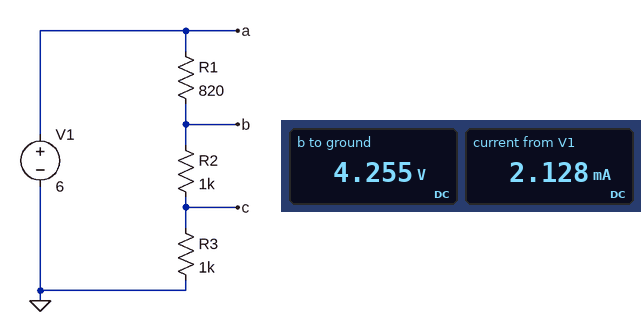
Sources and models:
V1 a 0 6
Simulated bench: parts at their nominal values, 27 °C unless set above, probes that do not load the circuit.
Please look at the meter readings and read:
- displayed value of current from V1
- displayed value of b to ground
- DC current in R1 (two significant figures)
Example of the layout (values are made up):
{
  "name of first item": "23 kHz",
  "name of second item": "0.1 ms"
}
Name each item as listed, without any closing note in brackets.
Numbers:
{
  "displayed value of current from V1": "2.128 mA",
  "displayed value of b to ground": "4.255 V",
  "DC current in R1": "2.1 mA"
}
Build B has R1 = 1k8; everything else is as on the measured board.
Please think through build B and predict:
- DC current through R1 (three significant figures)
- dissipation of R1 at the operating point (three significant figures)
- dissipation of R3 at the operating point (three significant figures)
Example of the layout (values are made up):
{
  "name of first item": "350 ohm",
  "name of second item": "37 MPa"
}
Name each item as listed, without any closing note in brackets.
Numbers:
{
  "DC current through R1": "1.58 mA",
  "dissipation of R1 at the operating point": "4.49 mW",
  "dissipation of R3 at the operating point": "2.49 mW"
}
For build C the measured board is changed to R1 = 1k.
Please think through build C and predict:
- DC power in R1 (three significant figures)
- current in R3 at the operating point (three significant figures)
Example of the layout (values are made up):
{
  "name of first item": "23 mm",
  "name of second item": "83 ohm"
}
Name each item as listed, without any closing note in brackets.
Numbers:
{
  "DC power in R1": "4.00 mW",
  "current in R3 at the operating point": "2.00 mA"
}
